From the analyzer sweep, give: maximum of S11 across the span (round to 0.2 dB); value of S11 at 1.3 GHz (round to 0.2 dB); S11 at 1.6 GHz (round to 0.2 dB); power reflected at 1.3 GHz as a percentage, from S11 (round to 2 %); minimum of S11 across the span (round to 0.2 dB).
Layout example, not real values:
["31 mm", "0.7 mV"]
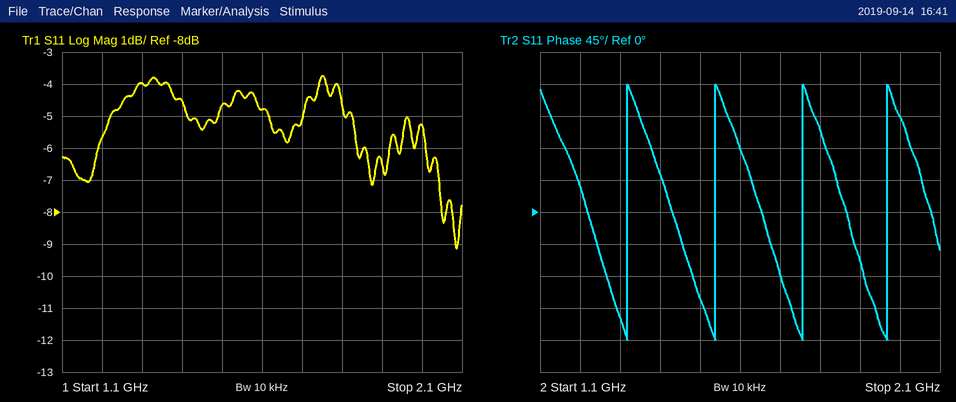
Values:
["-3.8 dB", "-4.0 dB", "-4.8 dB", "40 %", "-9.2 dB"]
